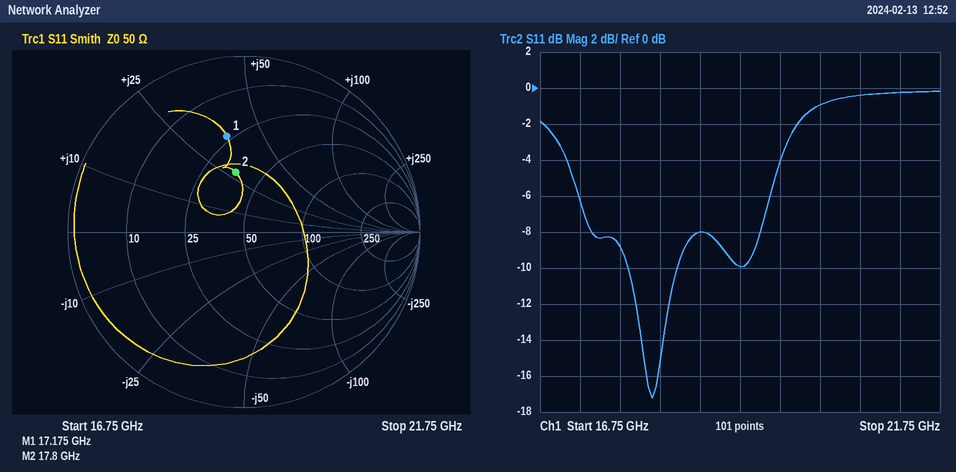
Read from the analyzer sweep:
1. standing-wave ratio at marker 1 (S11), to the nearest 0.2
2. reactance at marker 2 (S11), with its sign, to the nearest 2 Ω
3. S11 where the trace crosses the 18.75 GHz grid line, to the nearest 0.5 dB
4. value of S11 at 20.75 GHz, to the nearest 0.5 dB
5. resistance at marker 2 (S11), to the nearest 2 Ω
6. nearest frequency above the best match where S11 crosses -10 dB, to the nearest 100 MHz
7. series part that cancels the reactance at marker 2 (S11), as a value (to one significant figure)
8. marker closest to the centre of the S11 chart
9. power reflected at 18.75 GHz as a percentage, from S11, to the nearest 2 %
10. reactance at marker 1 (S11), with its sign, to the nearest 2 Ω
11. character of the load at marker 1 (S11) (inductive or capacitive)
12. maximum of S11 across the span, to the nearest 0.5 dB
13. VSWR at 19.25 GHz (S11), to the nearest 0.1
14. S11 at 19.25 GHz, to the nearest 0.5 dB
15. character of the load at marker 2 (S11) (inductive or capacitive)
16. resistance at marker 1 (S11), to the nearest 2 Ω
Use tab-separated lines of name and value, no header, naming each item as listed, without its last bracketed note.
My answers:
standing-wave ratio at marker 1 (S11), to the nearest 0.2	3.4
reactance at marker 2 (S11), with its sign, to the nearest 2 Ω	+28 Ω
S11 where the trace crosses the 18.75 GHz grid line, to the nearest 0.5 dB	-8.0 dB
value of S11 at 20.75 GHz, to the nearest 0.5 dB	-0.5 dB
resistance at marker 2 (S11), to the nearest 2 Ω	36 Ω
nearest frequency above the best match where S11 crosses -10 dB, to the nearest 100 MHz	18.5 GHz
series part that cancels the reactance at marker 2 (S11), as a value	300 fF
marker closest to the centre of the S11 chart	marker 2
power reflected at 18.75 GHz as a percentage, from S11, to the nearest 2 %	16 %
reactance at marker 1 (S11), with its sign, to the nearest 2 Ω	+36 Ω
character of the load at marker 1 (S11)	inductive
maximum of S11 across the span, to the nearest 0.5 dB	0.0 dB
VSWR at 19.25 GHz (S11), to the nearest 0.1	1.9
S11 at 19.25 GHz, to the nearest 0.5 dB	-10.0 dB
character of the load at marker 2 (S11)	inductive
resistance at marker 1 (S11), to the nearest 2 Ω	24 Ω
